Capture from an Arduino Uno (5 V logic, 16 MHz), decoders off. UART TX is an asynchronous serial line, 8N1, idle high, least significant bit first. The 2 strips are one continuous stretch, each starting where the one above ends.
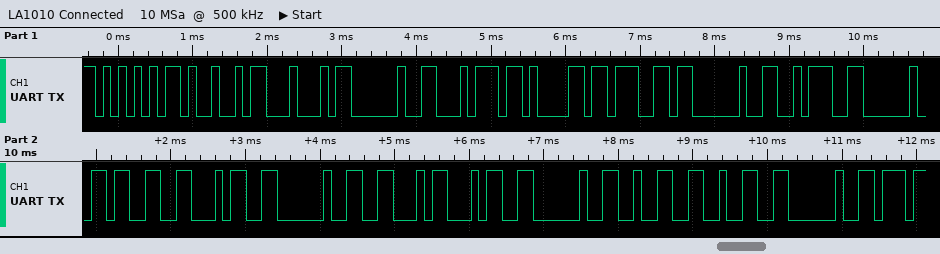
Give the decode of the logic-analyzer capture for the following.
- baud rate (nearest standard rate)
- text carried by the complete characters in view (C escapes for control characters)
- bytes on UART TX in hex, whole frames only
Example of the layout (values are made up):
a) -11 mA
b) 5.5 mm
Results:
a) 9600 baud
b) "UID tag : 34 F4 22 "
c) 55 49 44 20 74 61 67 20 3A 20 33 34 20 46 34 20 32 32 20
